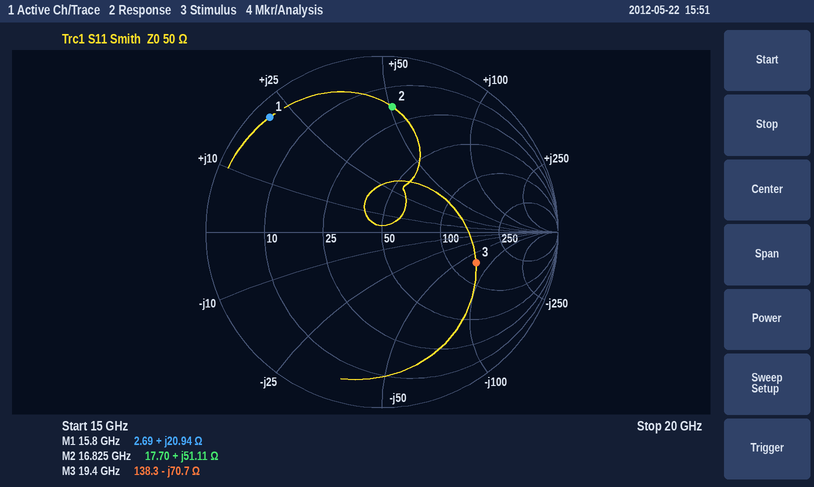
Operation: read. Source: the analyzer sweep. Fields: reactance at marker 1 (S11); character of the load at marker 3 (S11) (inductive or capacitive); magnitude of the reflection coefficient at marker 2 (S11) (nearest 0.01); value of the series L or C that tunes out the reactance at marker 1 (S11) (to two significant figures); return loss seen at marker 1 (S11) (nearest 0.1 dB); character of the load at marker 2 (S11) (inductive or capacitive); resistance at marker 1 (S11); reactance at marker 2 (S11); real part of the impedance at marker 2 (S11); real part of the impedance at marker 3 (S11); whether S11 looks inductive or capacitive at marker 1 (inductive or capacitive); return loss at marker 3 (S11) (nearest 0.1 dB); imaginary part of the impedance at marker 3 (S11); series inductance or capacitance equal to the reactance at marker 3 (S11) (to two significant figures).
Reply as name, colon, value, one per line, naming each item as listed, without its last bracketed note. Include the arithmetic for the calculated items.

reactance at marker 1: +20.94 Ω
character of the load at marker 3 (S11): capacitive
magnitude of the reflection coefficient at marker 2 (S11): 0.71
value of the series L or C that tunes out the reactance at marker 1 (S11): C = 1/(2π × 15.8 GHz × 20.94 Ω) ≈ 481 fF, so 480 fF to two significant figures
return loss seen at marker 1 (S11): 0.8 dB
character of the load at marker 2 (S11): inductive
resistance at marker 1: 2.69 Ω
reactance at marker 2: +51.11 Ω
real part of the impedance at marker 2: 17.70 Ω
real part of the impedance at marker 3: 138.3 Ω
whether S11 looks inductive or capacitive at marker 1: inductive
return loss at marker 3 (S11): 5.0 dB
imaginary part of the impedance at marker 3: -70.7 Ω
series inductance or capacitance equal to the reactance at marker 3 (S11): C = 1/(2π × 19.4 GHz × 70.7 Ω) ≈ 116 fF, so 120 fF to two significant figures
